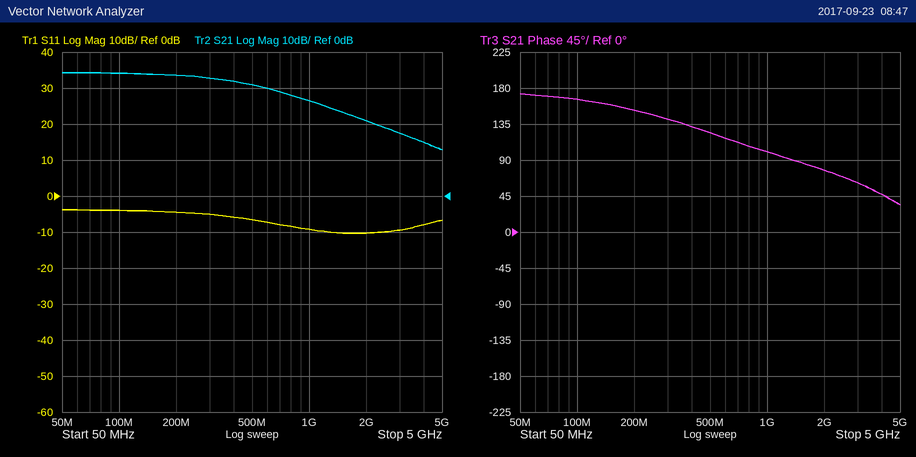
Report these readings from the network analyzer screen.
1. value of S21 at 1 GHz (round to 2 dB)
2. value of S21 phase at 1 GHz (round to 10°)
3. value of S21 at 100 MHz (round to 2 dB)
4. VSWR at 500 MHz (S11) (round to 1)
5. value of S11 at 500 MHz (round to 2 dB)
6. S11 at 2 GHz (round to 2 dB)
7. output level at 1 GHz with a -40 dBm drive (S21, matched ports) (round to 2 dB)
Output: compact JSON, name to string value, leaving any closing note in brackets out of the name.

{"value of S21 at 1 GHz": "26 dB", "value of S21 phase at 1 GHz": "100°", "value of S21 at 100 MHz": "34 dB", "VSWR at 500 MHz (S11)": "3", "value of S11 at 500 MHz": "-6 dB", "S11 at 2 GHz": "-10 dB", "output level at 1 GHz with a -40 dBm drive (S21, matched ports)": "-14 dBm"}
